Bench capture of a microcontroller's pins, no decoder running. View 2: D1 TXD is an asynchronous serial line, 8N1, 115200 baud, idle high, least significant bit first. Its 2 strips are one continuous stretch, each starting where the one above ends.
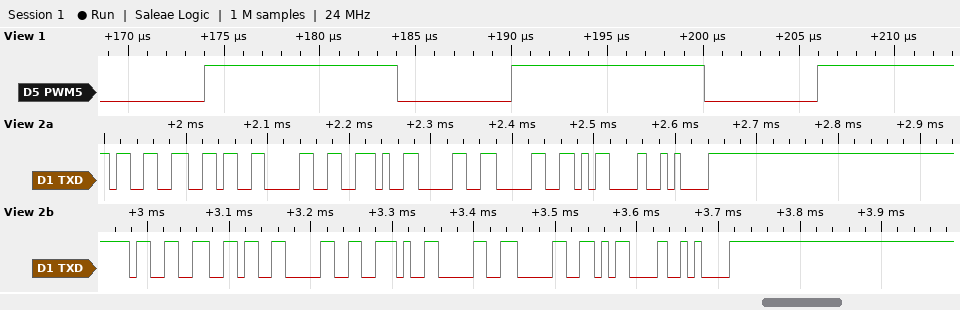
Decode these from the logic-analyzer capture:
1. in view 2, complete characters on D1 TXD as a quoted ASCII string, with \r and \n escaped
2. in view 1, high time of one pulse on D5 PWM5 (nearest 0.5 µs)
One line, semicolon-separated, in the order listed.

"360.00\r\n360.00\r\n"; 10.0 µs
